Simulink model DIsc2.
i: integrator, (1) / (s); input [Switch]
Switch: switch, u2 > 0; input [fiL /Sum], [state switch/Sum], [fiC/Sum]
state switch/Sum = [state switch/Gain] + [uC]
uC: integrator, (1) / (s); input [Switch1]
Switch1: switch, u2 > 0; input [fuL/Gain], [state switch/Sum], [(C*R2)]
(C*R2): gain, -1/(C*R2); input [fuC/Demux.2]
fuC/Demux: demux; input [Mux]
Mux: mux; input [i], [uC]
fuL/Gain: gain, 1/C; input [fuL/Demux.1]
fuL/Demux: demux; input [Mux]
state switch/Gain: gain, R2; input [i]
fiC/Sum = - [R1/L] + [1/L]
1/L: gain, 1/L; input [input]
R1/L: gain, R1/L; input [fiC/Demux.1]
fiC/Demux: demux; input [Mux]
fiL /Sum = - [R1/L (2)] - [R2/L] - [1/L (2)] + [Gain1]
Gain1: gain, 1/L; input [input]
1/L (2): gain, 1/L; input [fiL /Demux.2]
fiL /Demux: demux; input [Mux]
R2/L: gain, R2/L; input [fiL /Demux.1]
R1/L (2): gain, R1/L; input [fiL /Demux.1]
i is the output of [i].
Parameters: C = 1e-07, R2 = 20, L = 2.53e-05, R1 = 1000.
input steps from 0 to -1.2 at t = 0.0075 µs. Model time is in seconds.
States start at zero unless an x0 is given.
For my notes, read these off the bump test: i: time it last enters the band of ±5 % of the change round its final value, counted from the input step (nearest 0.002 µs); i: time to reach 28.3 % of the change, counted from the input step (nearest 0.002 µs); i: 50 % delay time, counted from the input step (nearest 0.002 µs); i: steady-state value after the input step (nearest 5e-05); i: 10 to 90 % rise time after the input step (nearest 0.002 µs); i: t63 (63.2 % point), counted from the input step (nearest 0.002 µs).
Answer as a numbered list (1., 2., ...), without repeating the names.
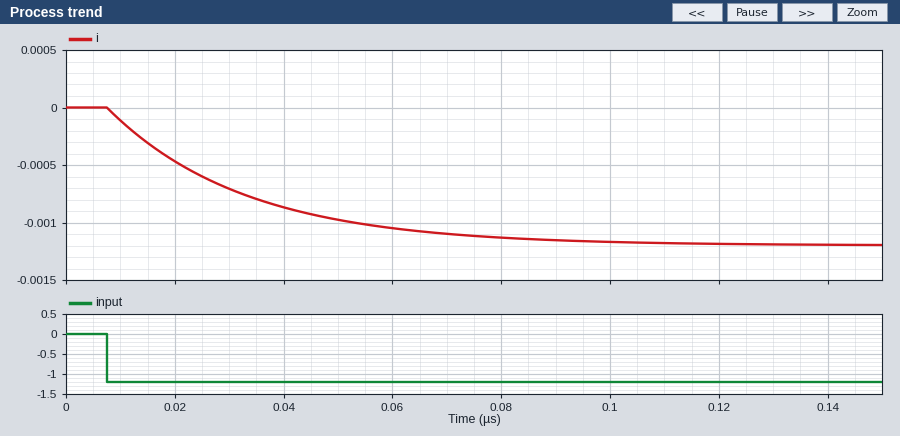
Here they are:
1. 0.076 µs
2. 0.008 µs
3. 0.018 µs
4. -0.00120
5. 0.056 µs
6. 0.026 µs
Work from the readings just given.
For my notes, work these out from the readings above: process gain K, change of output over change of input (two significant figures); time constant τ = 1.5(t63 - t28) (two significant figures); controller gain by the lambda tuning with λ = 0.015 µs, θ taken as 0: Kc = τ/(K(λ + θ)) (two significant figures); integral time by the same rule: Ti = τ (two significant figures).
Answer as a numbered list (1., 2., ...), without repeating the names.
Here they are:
1. 0.0010
2. 0.027 µs
3. 1800
4. 0.027 µs
